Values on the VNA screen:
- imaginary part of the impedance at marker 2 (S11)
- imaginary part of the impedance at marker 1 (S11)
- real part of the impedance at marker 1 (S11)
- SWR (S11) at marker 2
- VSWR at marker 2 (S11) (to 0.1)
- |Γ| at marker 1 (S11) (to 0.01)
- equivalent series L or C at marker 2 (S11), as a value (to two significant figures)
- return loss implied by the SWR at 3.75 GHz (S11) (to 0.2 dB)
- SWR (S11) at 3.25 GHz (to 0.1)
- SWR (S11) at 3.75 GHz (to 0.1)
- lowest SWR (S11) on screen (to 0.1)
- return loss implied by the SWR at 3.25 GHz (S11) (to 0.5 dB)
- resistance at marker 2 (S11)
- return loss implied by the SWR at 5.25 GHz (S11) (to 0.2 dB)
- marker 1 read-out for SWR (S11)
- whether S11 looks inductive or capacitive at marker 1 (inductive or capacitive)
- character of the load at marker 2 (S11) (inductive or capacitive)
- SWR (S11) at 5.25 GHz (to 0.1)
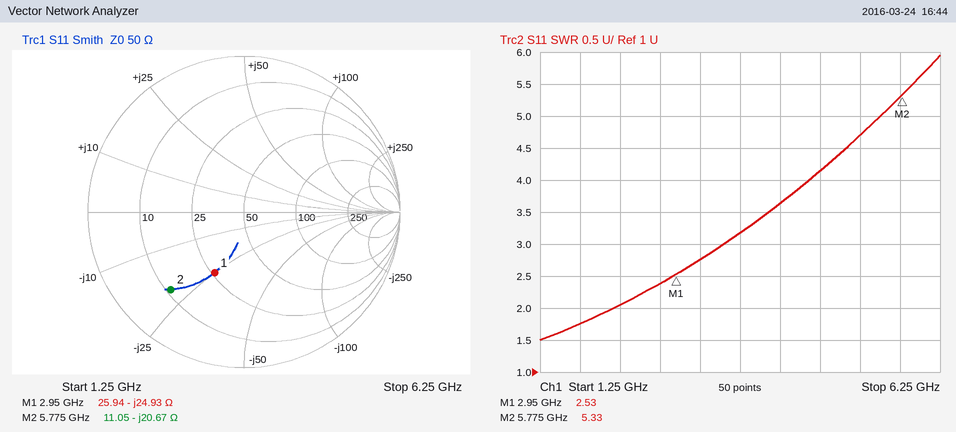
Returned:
-20.67 Ω
-24.93 Ω
25.94 Ω
5.33
5.3
0.43
1.3 pF
5.6 dB
2.8
3.2
1.5
6.5 dB
11.05 Ω
3.8 dB
2.53
capacitive
capacitive
4.7
